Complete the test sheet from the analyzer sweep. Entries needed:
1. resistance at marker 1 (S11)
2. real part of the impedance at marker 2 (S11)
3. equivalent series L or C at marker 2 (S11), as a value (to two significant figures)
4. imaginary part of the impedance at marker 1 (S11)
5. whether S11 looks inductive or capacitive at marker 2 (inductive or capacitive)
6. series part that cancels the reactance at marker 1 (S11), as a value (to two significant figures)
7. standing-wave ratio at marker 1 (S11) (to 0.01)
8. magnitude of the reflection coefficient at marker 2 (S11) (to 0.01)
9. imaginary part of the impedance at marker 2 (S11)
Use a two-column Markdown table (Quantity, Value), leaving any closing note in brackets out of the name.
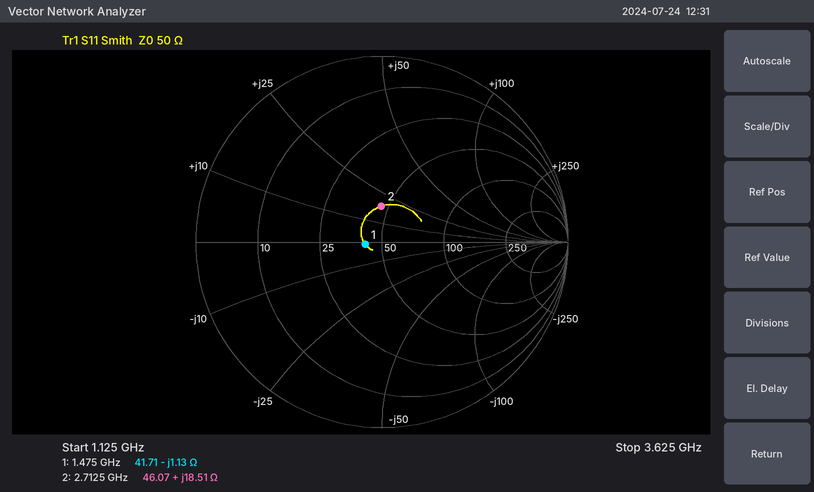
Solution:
| Quantity | Value |
|---|---|
| resistance at marker 1 | 41.71 Ω |
| real part of the impedance at marker 2 | 46.07 Ω |
| equivalent series L or C at marker 2 (S11), as a value | 1.1 nH |
| imaginary part of the impedance at marker 1 | -1.13 Ω |
| whether S11 looks inductive or capacitive at marker 2 | inductive |
| series part that cancels the reactance at marker 1 (S11), as a value | 120 pH |
| standing-wave ratio at marker 1 (S11) | 1.20 |
| magnitude of the reflection coefficient at marker 2 (S11) | 0.19 |
| imaginary part of the impedance at marker 2 | +18.51 Ω |
